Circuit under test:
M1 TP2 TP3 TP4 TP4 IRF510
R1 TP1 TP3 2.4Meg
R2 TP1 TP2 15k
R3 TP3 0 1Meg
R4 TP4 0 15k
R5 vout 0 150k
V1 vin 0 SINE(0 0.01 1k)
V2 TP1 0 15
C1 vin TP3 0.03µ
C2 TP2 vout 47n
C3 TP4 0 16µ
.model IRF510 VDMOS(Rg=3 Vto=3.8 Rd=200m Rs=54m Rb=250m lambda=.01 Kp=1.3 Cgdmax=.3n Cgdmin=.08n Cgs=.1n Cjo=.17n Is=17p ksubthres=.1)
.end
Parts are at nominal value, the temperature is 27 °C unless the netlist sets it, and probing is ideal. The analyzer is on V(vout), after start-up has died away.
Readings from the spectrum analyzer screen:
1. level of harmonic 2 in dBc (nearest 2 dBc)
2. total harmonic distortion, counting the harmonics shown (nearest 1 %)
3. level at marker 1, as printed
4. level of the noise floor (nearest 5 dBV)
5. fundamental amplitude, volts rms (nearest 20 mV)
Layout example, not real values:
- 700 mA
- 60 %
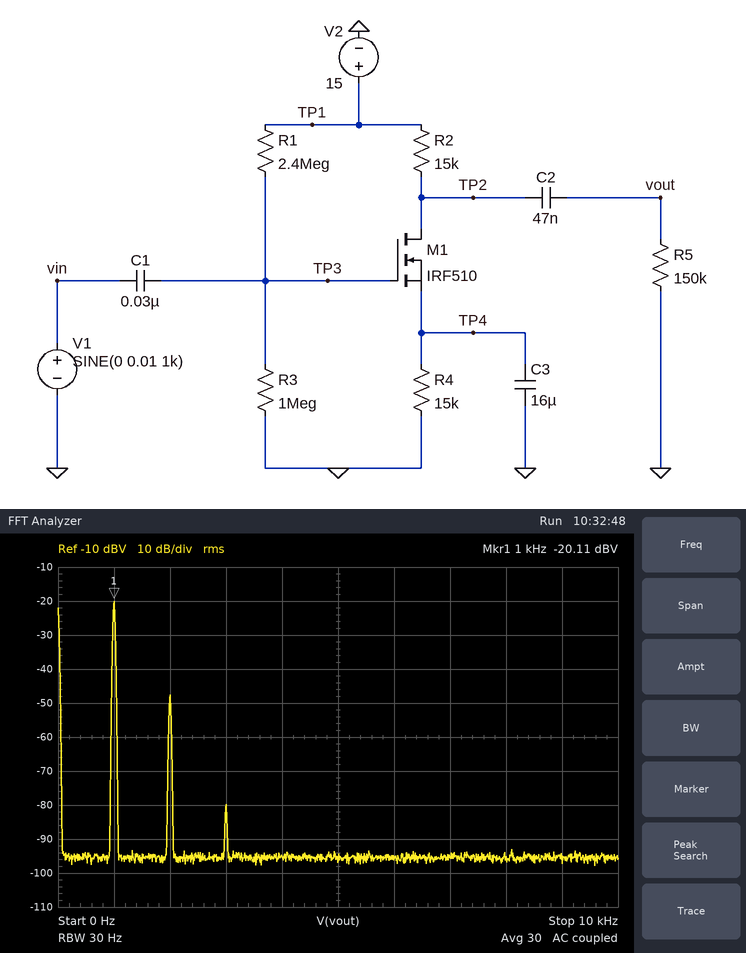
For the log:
- -28 dBc
- 4 %
- -20.11 dBV
- -95 dBV
- 100 mV
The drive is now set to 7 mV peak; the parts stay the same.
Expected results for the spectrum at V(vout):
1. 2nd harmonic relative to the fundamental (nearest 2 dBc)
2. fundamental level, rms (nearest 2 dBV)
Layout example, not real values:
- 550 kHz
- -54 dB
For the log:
- -30 dBc
- -24 dBV
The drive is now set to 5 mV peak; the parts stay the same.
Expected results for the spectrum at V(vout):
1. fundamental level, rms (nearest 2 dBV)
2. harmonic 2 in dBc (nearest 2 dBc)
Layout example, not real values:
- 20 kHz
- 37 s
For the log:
- -26 dBV
- -34 dBc
